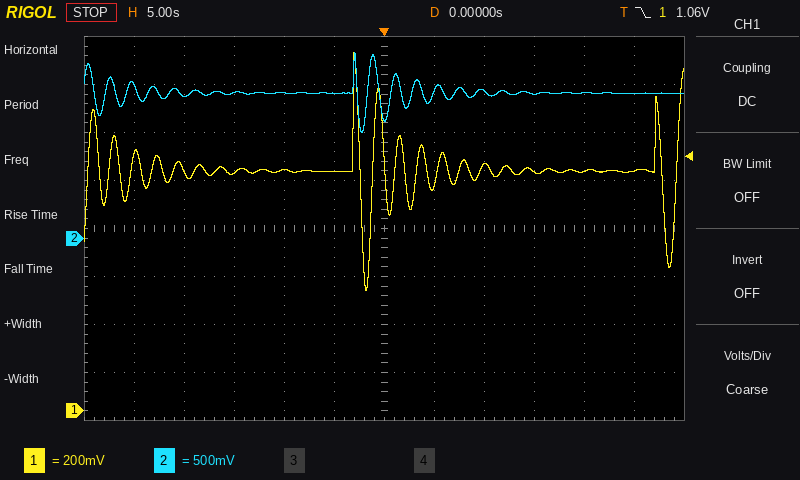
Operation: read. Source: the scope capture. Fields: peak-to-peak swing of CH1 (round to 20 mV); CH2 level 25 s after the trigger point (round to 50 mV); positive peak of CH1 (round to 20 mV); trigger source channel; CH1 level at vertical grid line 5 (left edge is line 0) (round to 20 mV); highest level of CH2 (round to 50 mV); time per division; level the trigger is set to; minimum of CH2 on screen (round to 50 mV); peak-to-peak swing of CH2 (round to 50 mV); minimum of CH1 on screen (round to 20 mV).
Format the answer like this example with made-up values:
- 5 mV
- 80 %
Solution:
- 1.00 V
- 1.50 V
- 1.50 V
- CH1
- 1.00 V
- 1.95 V
- 5 s
- 1.06 V
- 1.10 V
- 850 mV
- 500 mV
